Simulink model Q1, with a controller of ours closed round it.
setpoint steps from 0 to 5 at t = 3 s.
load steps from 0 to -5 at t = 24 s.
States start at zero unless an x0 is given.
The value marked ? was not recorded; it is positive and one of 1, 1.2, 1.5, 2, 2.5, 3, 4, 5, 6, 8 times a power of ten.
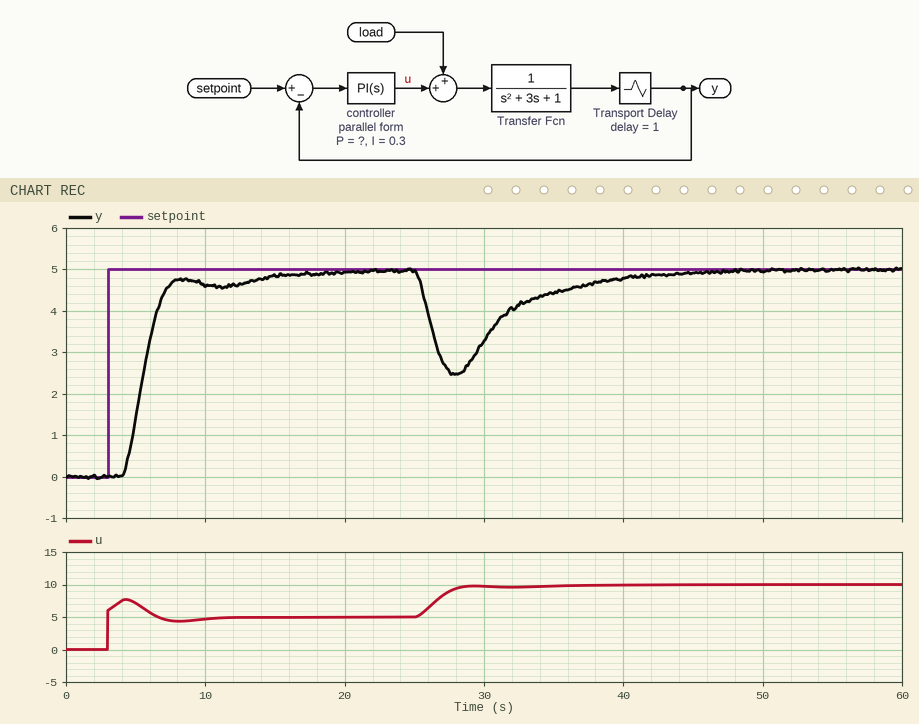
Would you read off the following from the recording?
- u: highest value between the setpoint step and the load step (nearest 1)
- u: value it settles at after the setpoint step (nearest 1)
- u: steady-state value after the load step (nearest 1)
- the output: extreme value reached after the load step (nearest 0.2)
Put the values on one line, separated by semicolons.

8; 5; 10; 2.4
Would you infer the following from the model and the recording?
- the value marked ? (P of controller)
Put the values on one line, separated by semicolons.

1.2
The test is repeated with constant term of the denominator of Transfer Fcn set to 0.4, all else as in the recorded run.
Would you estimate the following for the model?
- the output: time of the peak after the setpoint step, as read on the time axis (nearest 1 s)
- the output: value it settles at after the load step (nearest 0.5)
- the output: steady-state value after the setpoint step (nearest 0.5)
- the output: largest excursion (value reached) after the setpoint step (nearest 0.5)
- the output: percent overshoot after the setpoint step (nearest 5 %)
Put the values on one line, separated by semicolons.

9 s; 5.0; 5.0; 6.5; 30 %
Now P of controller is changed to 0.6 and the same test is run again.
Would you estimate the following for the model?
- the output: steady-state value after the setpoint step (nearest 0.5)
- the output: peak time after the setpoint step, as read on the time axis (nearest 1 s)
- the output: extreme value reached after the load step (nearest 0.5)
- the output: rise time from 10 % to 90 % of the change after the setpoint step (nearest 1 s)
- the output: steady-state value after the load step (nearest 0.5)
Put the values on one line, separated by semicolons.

5.0; 13 s; 2.0; 4 s; 5.0
